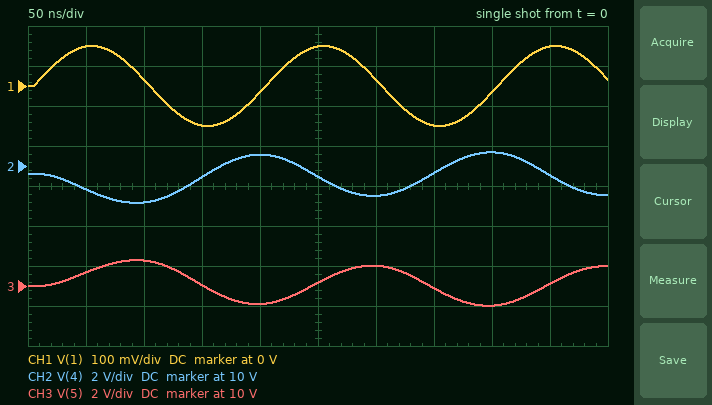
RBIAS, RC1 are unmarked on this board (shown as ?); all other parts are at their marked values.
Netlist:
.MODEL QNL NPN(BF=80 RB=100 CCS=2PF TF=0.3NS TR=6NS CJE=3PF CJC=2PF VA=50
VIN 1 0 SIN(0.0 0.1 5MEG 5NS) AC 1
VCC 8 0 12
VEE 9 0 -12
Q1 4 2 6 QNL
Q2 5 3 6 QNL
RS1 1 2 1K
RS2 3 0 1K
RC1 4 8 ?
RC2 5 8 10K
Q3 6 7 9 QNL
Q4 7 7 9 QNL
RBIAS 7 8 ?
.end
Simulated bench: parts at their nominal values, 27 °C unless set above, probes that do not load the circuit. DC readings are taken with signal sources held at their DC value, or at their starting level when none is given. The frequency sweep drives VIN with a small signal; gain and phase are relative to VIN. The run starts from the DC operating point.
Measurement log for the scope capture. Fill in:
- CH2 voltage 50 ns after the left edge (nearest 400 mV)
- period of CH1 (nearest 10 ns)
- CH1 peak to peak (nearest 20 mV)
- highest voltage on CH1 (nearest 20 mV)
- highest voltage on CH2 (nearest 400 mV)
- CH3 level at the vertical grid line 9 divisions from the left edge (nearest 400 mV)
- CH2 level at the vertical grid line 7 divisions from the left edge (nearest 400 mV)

8.8 V
200 ns
200 mV
100 mV
10.8 V
10.0 V
9.6 V
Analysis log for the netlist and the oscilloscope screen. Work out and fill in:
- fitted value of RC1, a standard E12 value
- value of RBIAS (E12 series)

12 kΩ
68 kΩ
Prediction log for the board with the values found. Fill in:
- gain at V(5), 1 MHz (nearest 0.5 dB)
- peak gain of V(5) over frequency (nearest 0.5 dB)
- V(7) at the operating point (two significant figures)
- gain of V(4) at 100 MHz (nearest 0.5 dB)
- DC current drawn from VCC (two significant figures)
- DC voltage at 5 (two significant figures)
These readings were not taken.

29.0 dB
30.5 dB
-11 V
-6.5 dB
740 µA
10 V
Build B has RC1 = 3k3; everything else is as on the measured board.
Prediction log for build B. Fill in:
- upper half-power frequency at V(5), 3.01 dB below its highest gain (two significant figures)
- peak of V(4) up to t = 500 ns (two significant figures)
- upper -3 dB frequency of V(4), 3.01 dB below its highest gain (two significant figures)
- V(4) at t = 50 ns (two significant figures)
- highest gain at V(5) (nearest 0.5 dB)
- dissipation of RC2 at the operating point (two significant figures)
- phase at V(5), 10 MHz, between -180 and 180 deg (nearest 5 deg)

2.2 MHz
12 V
2.5 MHz
11 V
31.0 dB
390 µW
-95 deg
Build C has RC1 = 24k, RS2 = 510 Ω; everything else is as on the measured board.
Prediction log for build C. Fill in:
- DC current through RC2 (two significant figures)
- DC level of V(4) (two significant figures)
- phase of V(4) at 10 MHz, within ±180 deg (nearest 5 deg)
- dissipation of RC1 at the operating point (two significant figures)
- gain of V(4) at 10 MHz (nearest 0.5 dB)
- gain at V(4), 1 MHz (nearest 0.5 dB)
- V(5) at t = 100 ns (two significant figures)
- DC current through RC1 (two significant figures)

210 µA
7.4 V
85 deg
880 µW
16.5 dB
35.0 dB
11 V
190 µA
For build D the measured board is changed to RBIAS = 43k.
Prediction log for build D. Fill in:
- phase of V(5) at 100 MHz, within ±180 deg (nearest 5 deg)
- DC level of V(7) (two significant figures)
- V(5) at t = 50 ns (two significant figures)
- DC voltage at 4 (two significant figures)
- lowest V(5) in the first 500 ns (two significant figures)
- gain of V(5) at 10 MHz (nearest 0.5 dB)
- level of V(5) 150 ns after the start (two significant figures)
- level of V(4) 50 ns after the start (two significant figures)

-155 deg
-11 V
9.6 V
8.2 V
7.7 V
15.5 dB
9.1 V
7.3 V
